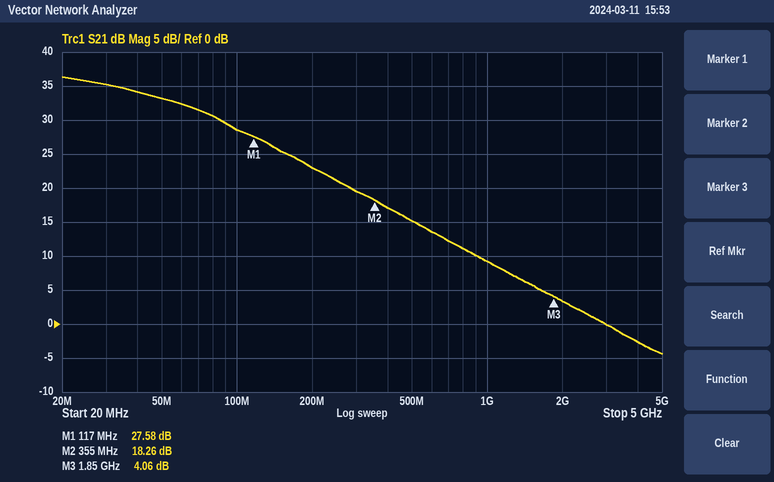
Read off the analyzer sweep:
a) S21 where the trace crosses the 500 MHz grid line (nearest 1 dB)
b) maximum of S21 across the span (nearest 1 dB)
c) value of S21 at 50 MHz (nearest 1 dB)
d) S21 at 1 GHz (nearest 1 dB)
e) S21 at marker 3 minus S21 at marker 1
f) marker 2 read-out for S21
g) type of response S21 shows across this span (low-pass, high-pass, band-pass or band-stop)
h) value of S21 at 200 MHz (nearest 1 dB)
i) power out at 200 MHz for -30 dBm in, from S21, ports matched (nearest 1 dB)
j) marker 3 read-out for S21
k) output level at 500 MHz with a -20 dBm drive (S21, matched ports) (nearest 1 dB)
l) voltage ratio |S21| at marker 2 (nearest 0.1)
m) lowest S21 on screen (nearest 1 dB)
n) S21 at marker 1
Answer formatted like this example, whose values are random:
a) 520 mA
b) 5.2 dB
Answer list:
a) 15 dB
b) 36 dB
c) 33 dB
d) 9 dB
e) -23.52 dB
f) 18.26 dB
g) low-pass
h) 23 dB
i) -7 dBm
j) 4.06 dB
k) -5 dBm
l) 8.2
m) -4 dB
n) 27.58 dB
